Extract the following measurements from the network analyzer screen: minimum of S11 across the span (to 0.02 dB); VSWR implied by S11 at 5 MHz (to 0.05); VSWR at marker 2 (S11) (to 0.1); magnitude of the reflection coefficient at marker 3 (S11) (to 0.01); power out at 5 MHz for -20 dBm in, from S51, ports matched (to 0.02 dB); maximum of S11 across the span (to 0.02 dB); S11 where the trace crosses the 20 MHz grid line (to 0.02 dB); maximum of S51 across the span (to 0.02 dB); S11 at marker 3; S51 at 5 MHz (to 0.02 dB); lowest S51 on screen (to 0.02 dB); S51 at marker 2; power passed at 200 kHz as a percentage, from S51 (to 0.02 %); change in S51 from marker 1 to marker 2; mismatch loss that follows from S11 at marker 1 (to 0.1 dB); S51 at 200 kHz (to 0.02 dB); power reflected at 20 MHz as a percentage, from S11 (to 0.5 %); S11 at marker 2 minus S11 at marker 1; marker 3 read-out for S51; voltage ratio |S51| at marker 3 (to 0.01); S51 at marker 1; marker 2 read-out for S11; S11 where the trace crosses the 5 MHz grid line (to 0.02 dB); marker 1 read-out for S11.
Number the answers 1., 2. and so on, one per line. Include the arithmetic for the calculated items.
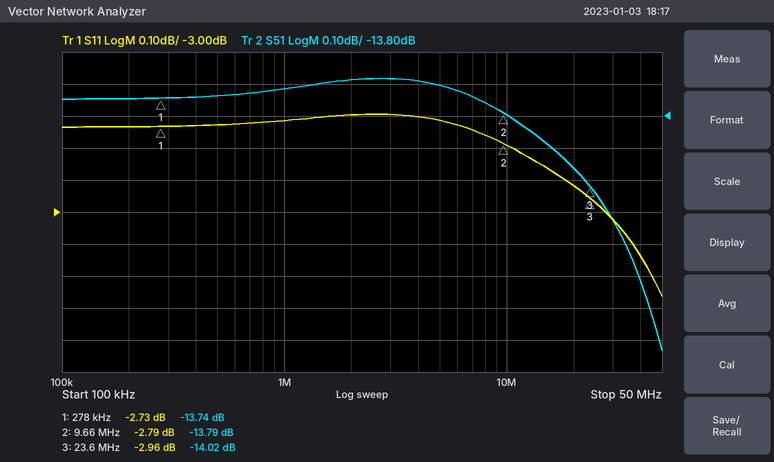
1. -3.26 dB
2. |Γ| = 10^(-2.72/20) = 0.7311; VSWR = (1 + 0.7311)/(1 − 0.7311) ≈ 6.44, so 6.45 to the nearest 0.05
3. (1 + 0.7253)/(1 − 0.7253) ≈ 6.3
4. 10^(-2.96/20) ≈ 0.71
5. -20 dBm + (-13.70 dB) = -33.70 dBm
6. -2.70 dB
7. -2.92 dB
8. -13.68 dB
9. -2.96 dB
10. -13.70 dB
11. -14.54 dB
12. -13.79 dB
13. 10^(-13.74/10) ≈ 4.23 %, so 4.22 % to the nearest 0.02 %
14. -13.79 − (-13.74) = -0.05 dB
15. −10 log10(1 − 10^(-2.73/10)) ≈ 3.3 dB
16. -13.74 dB
17. 10^(-2.92/10) ≈ 51.1 %, so 51.0 % to the nearest 0.5 %
18. -2.79 − (-2.73) = -0.06 dB
19. -14.02 dB
20. 10^(-14.02/20) ≈ 0.20
21. -13.74 dB
22. -2.79 dB
23. -2.72 dB
24. -2.73 dB
